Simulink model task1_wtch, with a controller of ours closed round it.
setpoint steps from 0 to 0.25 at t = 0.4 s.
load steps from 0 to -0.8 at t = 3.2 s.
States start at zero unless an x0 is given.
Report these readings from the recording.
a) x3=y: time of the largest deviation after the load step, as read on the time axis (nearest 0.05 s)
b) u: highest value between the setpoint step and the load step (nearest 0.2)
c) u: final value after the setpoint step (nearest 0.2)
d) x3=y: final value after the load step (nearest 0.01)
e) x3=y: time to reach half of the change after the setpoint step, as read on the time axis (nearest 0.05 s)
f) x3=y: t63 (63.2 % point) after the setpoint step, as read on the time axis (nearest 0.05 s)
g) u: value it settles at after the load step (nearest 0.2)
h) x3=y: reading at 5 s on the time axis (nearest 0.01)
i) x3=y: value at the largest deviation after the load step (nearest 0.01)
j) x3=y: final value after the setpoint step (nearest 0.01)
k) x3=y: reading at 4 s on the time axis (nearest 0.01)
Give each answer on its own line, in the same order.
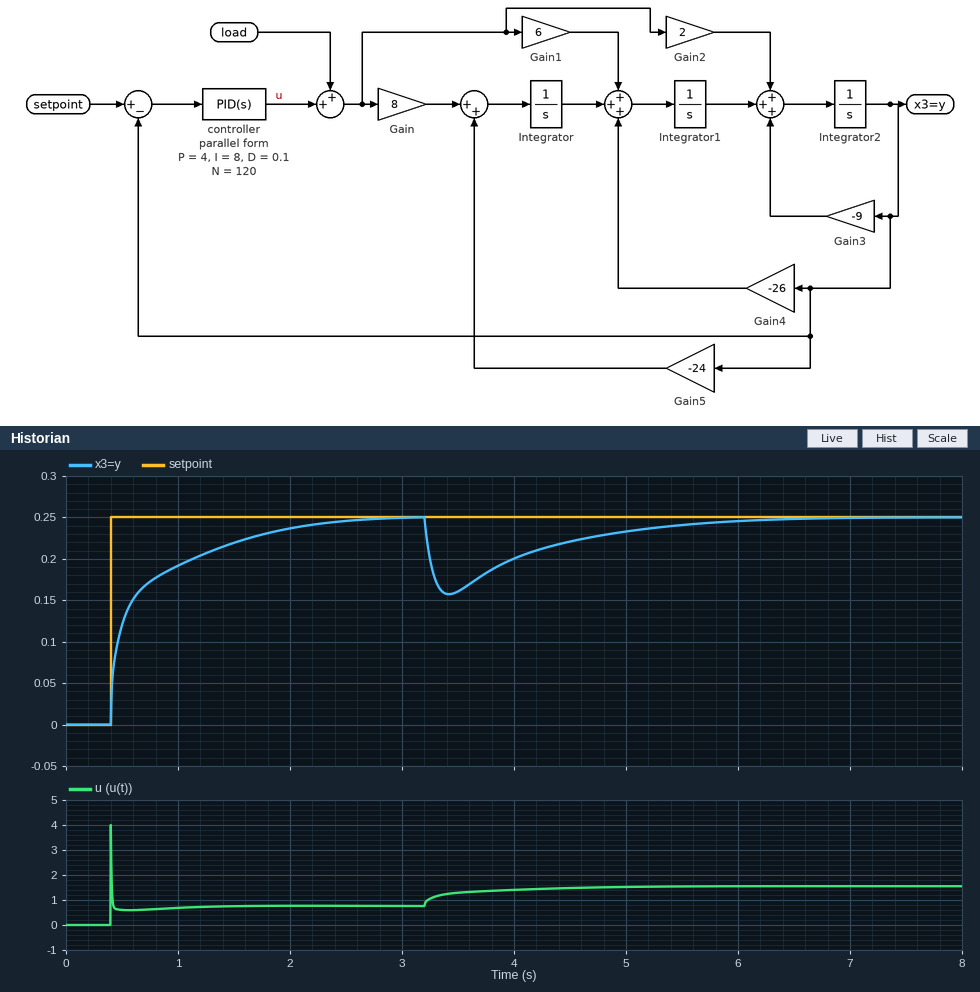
3.40 s
4.0
0.8
0.25
0.50 s
0.65 s
1.6
0.23
0.16
0.25
0.20
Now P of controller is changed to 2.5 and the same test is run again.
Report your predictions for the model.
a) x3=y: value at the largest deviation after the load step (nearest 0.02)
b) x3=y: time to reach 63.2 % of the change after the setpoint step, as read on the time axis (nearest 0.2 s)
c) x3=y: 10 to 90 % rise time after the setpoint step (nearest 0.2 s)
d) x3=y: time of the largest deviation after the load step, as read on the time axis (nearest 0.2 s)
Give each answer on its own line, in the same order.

0.14
0.8 s
1.2 s
3.4 s
